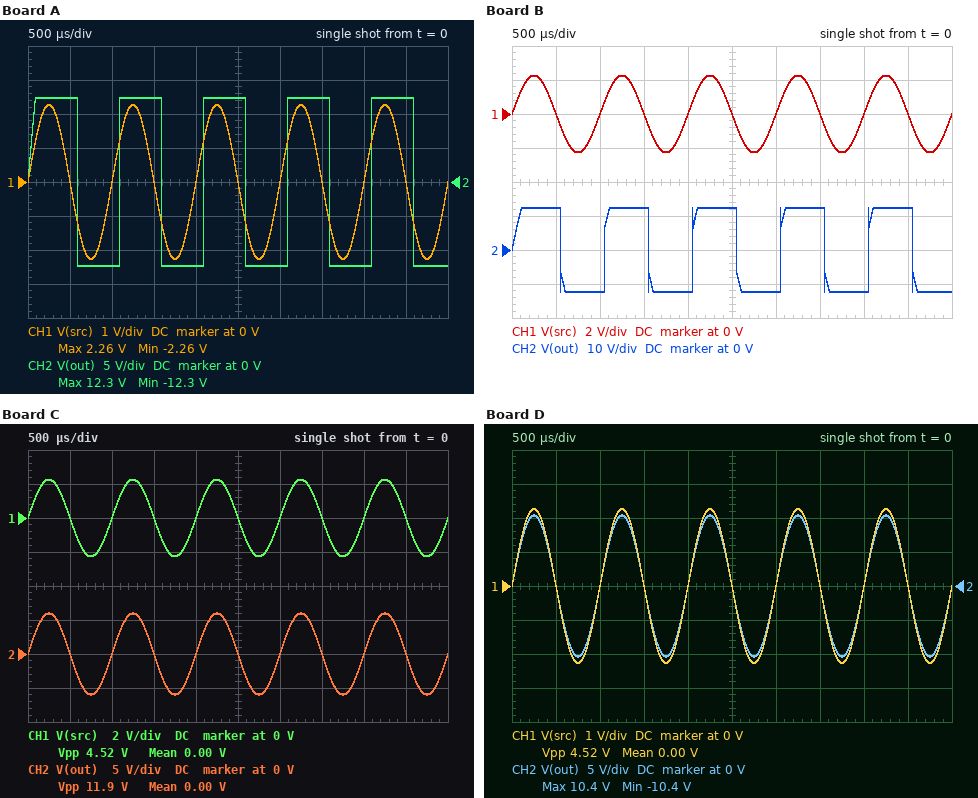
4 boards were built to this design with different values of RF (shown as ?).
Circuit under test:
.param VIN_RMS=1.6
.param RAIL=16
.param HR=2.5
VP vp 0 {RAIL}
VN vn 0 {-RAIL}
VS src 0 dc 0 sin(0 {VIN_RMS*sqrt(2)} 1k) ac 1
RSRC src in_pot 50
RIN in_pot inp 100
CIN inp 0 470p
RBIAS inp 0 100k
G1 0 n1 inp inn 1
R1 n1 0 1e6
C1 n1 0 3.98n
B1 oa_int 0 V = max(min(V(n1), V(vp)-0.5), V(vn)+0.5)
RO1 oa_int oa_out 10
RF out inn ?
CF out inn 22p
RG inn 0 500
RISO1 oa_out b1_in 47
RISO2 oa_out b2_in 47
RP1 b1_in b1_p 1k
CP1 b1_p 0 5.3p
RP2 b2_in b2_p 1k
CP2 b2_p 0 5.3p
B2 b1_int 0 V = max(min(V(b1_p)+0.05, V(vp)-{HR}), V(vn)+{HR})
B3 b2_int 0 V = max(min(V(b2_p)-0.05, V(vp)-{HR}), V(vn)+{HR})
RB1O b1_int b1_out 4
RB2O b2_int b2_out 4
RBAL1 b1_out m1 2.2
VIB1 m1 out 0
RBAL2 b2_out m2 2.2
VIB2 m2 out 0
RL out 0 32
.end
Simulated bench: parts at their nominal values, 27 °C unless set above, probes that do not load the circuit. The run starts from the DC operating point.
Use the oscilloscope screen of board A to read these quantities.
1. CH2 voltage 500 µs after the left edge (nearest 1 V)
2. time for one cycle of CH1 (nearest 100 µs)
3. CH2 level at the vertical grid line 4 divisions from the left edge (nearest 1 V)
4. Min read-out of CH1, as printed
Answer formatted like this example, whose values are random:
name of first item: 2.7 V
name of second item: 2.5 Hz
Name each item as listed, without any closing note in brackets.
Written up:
CH2 voltage 500 µs after the left edge: 12 V
time for one cycle of CH1: 1.0 ms
CH2 level at the vertical grid line 4 divisions from the left edge: -12 V
Min read-out of CH1, as printed: -2.26 V
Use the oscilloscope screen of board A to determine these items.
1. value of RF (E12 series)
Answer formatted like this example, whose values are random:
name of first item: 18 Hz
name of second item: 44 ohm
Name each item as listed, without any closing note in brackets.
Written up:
value of RF: 4.7 kΩ
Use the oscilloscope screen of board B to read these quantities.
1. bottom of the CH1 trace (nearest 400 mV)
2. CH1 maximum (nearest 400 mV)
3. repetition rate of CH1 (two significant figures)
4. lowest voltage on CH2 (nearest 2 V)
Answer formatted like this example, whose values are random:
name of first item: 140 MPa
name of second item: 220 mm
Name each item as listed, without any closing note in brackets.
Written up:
bottom of the CH1 trace: -2.4 V
CH1 maximum: 2.4 V
repetition rate of CH1: 1.0 kHz
lowest voltage on CH2: -12 V
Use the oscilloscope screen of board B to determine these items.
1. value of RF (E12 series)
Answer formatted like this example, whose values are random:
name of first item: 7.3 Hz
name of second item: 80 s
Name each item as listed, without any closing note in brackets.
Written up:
value of RF: 3.9 kΩ
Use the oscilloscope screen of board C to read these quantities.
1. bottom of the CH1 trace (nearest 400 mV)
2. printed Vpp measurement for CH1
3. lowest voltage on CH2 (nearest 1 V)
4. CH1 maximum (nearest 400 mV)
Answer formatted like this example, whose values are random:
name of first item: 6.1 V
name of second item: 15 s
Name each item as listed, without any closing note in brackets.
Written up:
bottom of the CH1 trace: -2.4 V
printed Vpp measurement for CH1: 4.52 V
lowest voltage on CH2: -6 V
CH1 maximum: 2.4 V
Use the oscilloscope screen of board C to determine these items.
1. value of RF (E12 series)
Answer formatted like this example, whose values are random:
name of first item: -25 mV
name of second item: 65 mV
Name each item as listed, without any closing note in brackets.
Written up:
value of RF: 820 Ω
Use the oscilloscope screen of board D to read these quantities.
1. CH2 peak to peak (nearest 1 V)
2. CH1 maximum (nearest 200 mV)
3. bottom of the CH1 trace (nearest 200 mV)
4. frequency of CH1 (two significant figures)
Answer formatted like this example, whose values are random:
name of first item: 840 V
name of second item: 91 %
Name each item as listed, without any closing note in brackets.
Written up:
CH2 peak to peak: 21 V
CH1 maximum: 2.2 V
bottom of the CH1 trace: -2.2 V
frequency of CH1: 1.0 kHz
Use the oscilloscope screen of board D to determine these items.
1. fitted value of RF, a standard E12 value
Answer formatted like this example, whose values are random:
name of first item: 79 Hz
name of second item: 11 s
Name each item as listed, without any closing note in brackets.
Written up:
fitted value of RF, a standard E12 value: 1.8 kΩ
